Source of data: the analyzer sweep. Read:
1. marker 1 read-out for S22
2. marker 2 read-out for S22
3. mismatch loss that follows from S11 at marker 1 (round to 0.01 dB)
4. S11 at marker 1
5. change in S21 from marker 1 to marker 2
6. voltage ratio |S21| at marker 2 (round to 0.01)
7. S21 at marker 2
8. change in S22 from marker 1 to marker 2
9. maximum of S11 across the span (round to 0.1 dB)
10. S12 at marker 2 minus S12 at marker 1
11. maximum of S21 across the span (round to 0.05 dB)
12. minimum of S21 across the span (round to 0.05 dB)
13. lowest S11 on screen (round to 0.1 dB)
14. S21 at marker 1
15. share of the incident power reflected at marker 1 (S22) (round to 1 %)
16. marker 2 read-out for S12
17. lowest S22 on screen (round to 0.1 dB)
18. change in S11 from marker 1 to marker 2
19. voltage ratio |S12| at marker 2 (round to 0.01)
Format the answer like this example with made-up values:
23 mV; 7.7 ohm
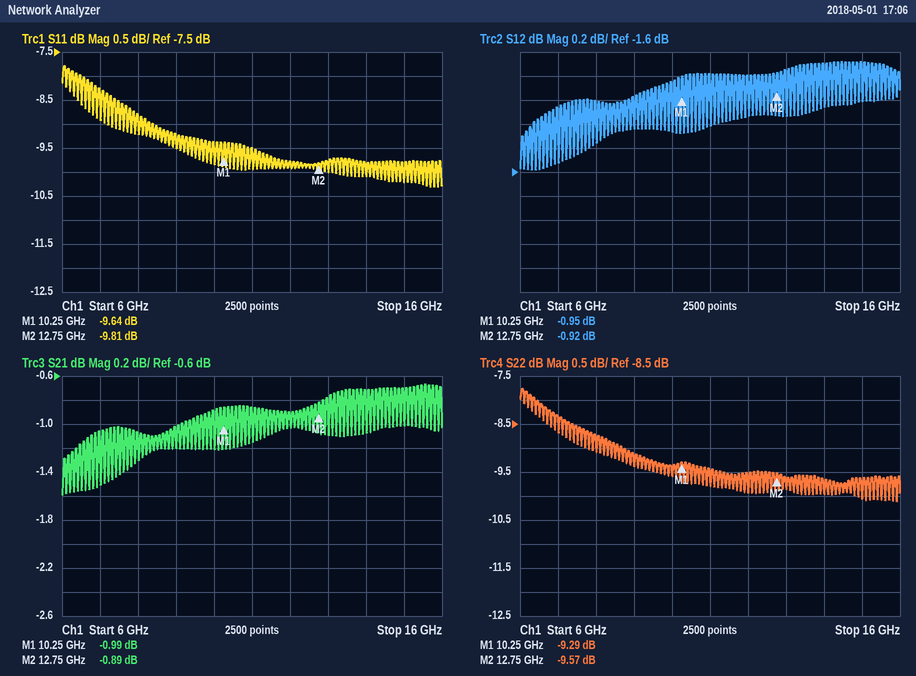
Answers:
-9.29 dB; -9.57 dB; 0.50 dB; -9.64 dB; 0.10 dB; 0.90; -0.89 dB; -0.28 dB; -7.8 dB; 0.03 dB; -0.65 dB; -1.60 dB; -10.3 dB; -0.99 dB; 12 %; -0.92 dB; -10.1 dB; -0.17 dB; 0.90
